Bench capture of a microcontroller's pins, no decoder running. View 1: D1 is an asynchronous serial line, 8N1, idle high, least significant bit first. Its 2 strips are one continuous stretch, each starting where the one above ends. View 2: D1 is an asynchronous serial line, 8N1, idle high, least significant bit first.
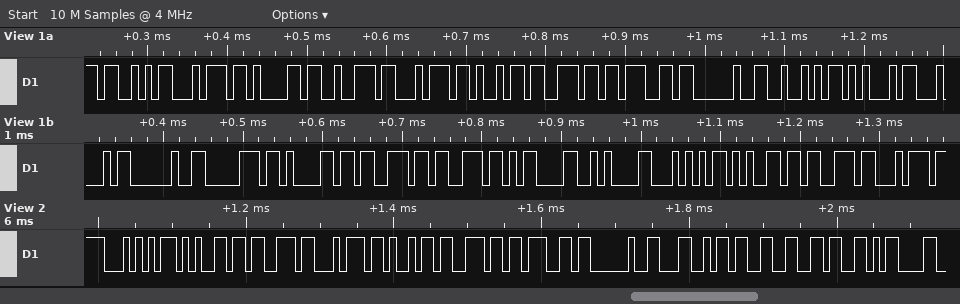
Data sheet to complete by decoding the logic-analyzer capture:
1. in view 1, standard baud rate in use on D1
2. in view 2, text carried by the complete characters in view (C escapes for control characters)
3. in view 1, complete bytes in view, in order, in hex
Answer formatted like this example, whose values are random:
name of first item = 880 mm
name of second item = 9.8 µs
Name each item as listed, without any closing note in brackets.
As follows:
in view 1, standard baud rate in use on D1 = 115200 baud
in view 2, text carried by the complete characters in view = "Testing L36\r"
in view 1, complete bytes in view, in order, in hex = 53 74 61 72 74 69 6E 67 20 52 45 44 20 70 61 73 73 0D 0A 54 65 73 74
